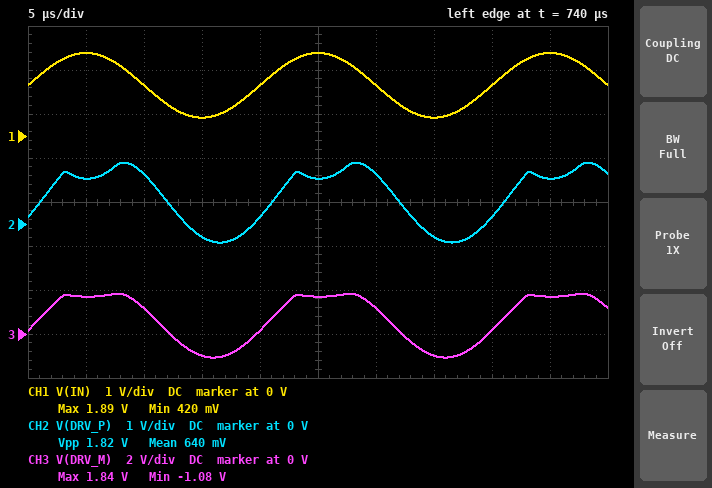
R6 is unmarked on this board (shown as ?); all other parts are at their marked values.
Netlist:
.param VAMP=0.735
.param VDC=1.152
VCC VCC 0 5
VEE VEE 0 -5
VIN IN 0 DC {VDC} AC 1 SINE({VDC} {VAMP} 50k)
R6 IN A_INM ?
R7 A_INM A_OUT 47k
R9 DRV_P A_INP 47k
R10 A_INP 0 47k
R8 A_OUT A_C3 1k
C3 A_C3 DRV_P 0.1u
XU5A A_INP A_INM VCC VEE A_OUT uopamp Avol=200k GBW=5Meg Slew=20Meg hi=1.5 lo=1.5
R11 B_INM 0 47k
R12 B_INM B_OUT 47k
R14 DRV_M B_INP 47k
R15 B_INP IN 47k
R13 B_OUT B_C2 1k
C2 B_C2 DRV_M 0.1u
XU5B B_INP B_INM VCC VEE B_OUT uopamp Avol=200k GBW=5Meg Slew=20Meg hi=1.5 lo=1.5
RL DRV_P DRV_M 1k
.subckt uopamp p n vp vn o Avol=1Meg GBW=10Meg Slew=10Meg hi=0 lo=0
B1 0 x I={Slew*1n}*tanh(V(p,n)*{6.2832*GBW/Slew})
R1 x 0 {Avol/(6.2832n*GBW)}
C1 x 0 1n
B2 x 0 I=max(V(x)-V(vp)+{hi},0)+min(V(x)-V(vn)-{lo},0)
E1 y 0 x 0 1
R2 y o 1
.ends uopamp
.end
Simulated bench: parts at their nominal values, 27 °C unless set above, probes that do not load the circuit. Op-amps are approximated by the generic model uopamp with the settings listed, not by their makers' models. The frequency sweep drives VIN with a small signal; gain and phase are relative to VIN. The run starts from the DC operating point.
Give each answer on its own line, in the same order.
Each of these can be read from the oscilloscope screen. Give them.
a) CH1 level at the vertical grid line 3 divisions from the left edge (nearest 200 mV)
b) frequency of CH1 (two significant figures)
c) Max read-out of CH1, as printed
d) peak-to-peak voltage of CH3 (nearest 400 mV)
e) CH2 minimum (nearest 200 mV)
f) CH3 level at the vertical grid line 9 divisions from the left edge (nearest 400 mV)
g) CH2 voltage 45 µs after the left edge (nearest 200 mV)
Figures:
400 mV
50 kHz
1.89 V
2.8 V
-400 mV
1.6 V
1.0 V
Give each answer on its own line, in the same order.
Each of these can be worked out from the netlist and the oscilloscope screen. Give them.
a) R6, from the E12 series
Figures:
56 kΩ
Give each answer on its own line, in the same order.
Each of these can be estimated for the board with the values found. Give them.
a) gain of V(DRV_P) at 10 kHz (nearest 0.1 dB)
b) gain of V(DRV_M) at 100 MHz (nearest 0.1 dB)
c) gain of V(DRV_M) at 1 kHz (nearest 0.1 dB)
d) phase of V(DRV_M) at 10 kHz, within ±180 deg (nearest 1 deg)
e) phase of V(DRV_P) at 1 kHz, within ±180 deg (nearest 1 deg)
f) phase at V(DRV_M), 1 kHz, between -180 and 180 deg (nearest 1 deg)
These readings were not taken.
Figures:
4.0 dB
-38.7 dB
5.6 dB
0 deg
12 deg
23 deg
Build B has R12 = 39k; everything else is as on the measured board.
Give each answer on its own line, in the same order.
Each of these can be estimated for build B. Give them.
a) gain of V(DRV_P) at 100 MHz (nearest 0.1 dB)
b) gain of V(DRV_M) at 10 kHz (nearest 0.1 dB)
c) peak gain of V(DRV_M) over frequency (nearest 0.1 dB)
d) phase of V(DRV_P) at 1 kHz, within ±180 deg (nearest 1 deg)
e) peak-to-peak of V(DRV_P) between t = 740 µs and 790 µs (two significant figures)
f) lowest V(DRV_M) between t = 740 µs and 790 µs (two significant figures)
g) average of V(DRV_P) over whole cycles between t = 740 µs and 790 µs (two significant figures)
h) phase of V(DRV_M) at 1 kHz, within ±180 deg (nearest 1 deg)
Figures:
-42.5 dB
-1.3 dB
-1.2 dB
-32 deg
130 mV
-53 mV
570 mV
17 deg
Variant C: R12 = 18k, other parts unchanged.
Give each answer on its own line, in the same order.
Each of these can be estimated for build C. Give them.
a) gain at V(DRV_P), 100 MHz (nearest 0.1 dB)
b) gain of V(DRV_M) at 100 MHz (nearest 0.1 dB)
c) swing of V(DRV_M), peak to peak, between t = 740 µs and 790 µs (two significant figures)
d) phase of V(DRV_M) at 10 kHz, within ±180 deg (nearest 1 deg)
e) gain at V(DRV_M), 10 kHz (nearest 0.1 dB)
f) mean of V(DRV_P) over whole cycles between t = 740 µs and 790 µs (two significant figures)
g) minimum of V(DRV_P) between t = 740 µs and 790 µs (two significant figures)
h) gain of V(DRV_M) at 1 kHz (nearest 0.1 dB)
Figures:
-42.4 dB
-38.6 dB
250 mV
171 deg
-15.3 dB
570 mV
-100 mV
-11.4 dB
